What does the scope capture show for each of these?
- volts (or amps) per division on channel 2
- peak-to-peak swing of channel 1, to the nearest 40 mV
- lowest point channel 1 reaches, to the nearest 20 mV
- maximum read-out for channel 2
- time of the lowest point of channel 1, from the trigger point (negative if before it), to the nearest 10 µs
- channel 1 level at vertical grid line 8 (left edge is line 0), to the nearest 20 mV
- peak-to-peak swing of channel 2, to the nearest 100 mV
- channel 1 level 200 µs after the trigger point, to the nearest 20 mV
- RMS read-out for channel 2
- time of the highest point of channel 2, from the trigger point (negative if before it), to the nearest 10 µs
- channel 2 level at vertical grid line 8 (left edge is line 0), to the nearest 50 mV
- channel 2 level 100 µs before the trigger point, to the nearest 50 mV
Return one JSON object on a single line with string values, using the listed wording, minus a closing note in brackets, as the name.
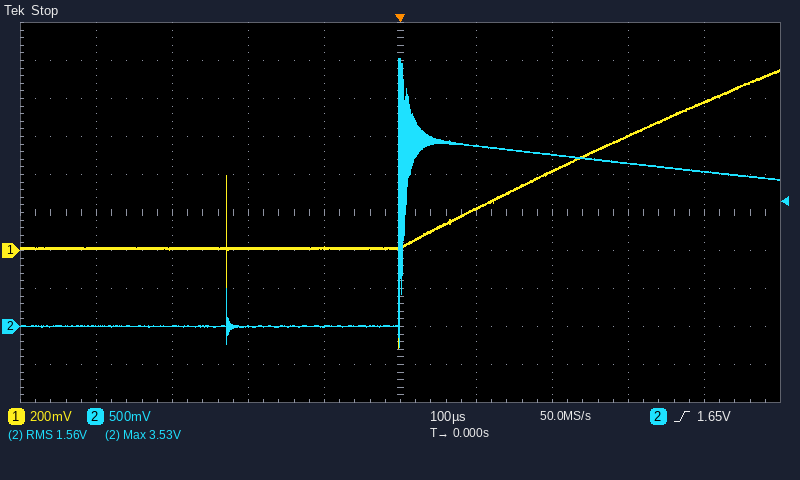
{"volts (or amps) per division on channel 2": "500 mV", "peak-to-peak swing of channel 1, to the nearest 40 mV": "1.48 V", "lowest point channel 1 reaches, to the nearest 20 mV": "-520 mV", "maximum read-out for channel 2": "3.53 V", "time of the lowest point of channel 1, from the trigger point (negative if before it), to the nearest 10 µs": "0 µs", "channel 1 level at vertical grid line 8 (left edge is line 0), to the nearest 20 mV": "600 mV", "peak-to-peak swing of channel 2, to the nearest 100 mV": "3.80 V", "channel 1 level 200 µs after the trigger point, to the nearest 20 mV": "420 mV", "RMS read-out for channel 2": "1.56 V", "time of the highest point of channel 2, from the trigger point (negative if before it), to the nearest 10 µs": "0 µs", "channel 2 level at vertical grid line 8 (left edge is line 0), to the nearest 50 mV": "2.15 V", "channel 2 level 100 µs before the trigger point, to the nearest 50 mV": "0 mV"}
